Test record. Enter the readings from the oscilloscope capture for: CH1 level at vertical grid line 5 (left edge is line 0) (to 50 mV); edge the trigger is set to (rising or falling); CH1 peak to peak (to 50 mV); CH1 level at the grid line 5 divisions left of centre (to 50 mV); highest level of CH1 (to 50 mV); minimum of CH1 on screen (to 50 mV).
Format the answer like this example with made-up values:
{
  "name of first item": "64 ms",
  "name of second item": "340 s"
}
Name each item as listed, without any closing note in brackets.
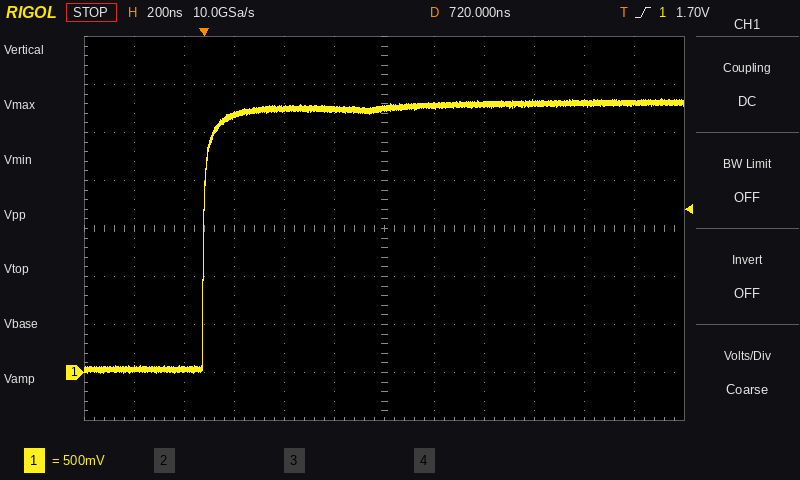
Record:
{
  "CH1 level at vertical grid line 5 (left edge is line 0)": "2.75 V",
  "edge the trigger is set to": "rising",
  "CH1 peak to peak": "2.85 V",
  "CH1 level at the grid line 5 divisions left of centre": "50 mV",
  "highest level of CH1": "2.85 V",
  "minimum of CH1 on screen": "0 mV"
}
